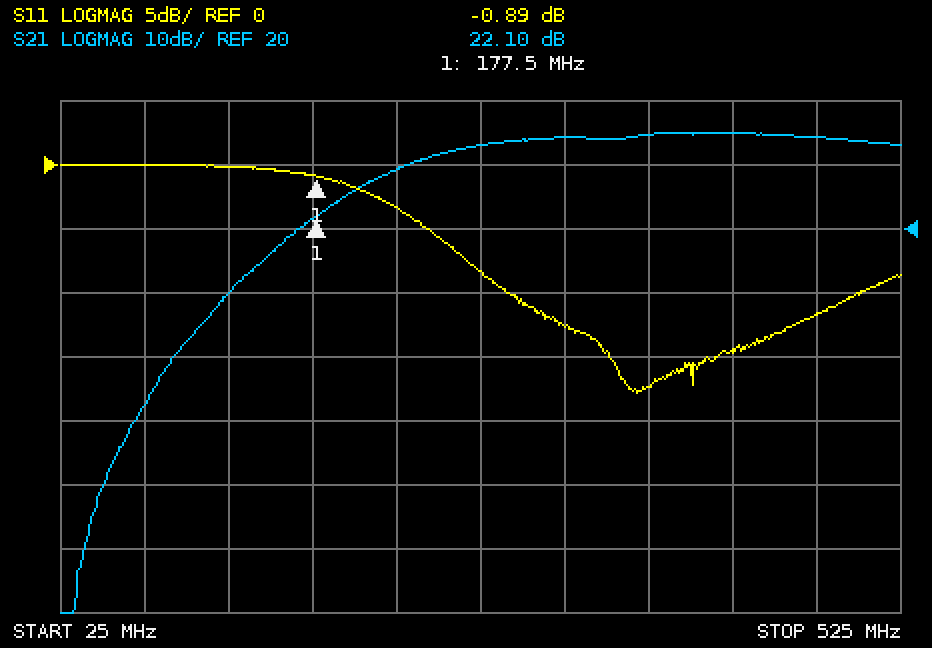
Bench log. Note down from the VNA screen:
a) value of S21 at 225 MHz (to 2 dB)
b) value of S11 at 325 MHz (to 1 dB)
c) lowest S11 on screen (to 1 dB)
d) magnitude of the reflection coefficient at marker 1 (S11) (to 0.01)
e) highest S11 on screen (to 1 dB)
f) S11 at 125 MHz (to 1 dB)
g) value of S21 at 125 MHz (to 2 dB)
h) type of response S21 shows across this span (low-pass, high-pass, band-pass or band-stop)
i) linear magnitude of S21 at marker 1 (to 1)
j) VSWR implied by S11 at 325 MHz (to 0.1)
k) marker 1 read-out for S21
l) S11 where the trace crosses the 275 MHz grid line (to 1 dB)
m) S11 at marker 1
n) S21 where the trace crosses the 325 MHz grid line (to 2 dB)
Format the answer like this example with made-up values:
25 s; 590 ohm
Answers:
30 dB; -13 dB; -18 dB; 0.90; 0 dB; 0 dB; 10 dB; high-pass; 13; 1.6; 22.10 dB; -8 dB; -0.89 dB; 34 dB
